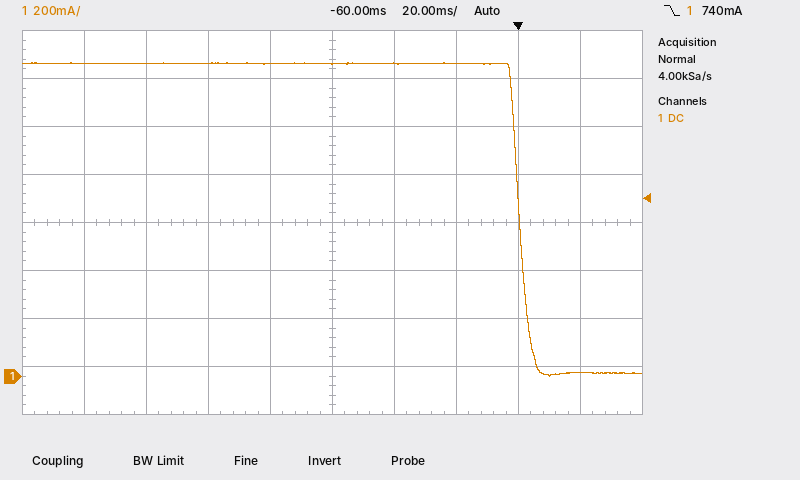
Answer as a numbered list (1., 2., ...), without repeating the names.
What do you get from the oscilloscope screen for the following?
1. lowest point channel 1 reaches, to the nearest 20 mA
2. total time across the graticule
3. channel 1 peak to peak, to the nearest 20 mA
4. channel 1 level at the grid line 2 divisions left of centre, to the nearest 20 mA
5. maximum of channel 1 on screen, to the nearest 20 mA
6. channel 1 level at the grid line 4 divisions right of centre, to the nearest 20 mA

1. 0 mA
2. 200 ms
3. 1.30 A
4. 1.30 A
5. 1.30 A
6. 20 mA
